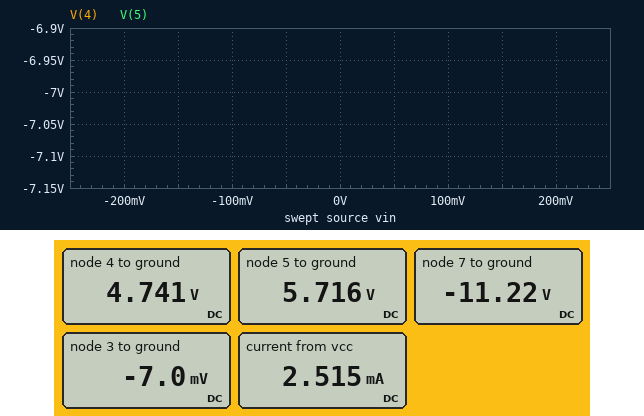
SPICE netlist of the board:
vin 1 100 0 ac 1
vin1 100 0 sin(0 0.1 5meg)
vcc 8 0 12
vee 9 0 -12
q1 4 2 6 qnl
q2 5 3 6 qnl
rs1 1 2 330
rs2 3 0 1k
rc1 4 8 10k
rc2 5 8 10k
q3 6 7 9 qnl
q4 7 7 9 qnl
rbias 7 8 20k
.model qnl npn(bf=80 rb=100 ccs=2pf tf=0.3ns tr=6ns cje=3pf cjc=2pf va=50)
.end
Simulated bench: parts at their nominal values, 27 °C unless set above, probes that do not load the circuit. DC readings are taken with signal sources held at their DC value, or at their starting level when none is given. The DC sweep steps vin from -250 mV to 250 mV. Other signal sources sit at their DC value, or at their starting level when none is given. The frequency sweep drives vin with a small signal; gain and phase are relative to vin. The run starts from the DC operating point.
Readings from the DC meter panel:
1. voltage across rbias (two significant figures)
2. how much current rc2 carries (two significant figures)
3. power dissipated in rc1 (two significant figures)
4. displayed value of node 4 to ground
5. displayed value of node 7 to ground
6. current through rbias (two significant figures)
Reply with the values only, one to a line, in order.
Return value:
23 V
630 µA
5.3 mW
4.741 V
-11.22 V
1.2 mA
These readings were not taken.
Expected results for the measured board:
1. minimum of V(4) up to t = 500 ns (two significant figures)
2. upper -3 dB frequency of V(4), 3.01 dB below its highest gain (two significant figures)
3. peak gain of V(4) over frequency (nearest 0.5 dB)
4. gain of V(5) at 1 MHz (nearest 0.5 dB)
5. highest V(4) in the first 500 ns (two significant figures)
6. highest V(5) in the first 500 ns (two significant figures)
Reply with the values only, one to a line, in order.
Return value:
2.2 V
890 kHz
39.5 dB
36.0 dB
6.2 V
8.3 V
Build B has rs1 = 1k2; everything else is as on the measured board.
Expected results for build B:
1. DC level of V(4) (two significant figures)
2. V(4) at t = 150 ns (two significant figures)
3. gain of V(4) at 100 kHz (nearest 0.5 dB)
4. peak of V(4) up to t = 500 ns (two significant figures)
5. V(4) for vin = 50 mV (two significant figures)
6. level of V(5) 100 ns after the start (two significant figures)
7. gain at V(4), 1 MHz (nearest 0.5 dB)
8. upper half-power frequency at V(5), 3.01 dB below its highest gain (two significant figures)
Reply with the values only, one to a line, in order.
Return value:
5.4 V
4.9 V
38.5 dB
6.2 V
1.4 V
6.9 V
33.5 dB
650 kHz
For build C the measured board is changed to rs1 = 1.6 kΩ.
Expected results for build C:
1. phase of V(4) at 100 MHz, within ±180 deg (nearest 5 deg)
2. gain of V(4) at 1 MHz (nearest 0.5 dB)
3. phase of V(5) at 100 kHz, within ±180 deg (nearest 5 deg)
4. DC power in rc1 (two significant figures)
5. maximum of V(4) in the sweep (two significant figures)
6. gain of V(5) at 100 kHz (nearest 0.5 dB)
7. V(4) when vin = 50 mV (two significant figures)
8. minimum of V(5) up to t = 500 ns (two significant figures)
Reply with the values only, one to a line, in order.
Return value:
45 deg
32.5 dB
-10 deg
4.1 mW
12 V
38.0 dB
1.7 V
4.1 V
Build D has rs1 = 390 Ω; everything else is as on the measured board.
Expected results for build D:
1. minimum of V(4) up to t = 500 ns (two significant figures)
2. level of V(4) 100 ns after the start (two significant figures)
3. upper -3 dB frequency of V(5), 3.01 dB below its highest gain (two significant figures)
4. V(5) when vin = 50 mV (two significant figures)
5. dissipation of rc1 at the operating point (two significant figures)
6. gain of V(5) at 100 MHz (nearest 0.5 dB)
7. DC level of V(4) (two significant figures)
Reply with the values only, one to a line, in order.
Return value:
2.3 V
2.4 V
870 kHz
9.7 V
5.2 mW
-6.0 dB
4.8 V
